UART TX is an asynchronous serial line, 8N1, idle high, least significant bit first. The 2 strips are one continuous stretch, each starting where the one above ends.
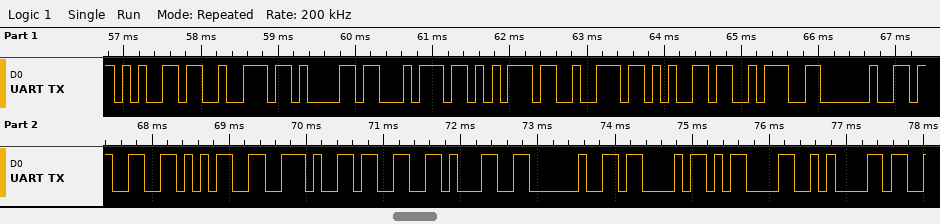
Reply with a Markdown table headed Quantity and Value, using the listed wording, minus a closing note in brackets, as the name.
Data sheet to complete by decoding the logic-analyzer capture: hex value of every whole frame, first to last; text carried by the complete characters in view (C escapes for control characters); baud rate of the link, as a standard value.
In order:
| Quantity | Value |
|---|---|
| hex value of every whole frame, first to last | 65 72 61 74 75 72 65 3A 20 33 35 2E 33 31 20 43 0D 0A |
| text carried by the complete characters in view | "erature: 35.31 C\r\n" |
| baud rate of the link, as a standard value | 9600 baud |
